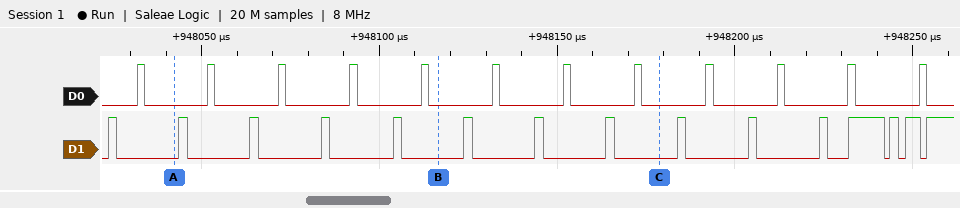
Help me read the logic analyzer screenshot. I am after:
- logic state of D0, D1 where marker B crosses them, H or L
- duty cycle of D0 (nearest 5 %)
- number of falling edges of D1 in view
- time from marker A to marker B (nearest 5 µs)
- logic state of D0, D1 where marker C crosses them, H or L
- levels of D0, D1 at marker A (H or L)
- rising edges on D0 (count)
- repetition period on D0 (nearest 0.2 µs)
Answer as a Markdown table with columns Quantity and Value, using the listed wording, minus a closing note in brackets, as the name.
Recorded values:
| Quantity | Value |
|---|---|
| logic state of D0, D1 where marker B crosses them, H or L | D0=L, D1=L |
| duty cycle of D0 | 10 % |
| number of falling edges of D1 in view | 14 |
| time from marker A to marker B | 75 µs |
| logic state of D0, D1 where marker C crosses them, H or L | D0=L, D1=L |
| levels of D0, D1 at marker A | D0=L, D1=L |
| rising edges on D0 | 12 |
| repetition period on D0 | 20 µs |
